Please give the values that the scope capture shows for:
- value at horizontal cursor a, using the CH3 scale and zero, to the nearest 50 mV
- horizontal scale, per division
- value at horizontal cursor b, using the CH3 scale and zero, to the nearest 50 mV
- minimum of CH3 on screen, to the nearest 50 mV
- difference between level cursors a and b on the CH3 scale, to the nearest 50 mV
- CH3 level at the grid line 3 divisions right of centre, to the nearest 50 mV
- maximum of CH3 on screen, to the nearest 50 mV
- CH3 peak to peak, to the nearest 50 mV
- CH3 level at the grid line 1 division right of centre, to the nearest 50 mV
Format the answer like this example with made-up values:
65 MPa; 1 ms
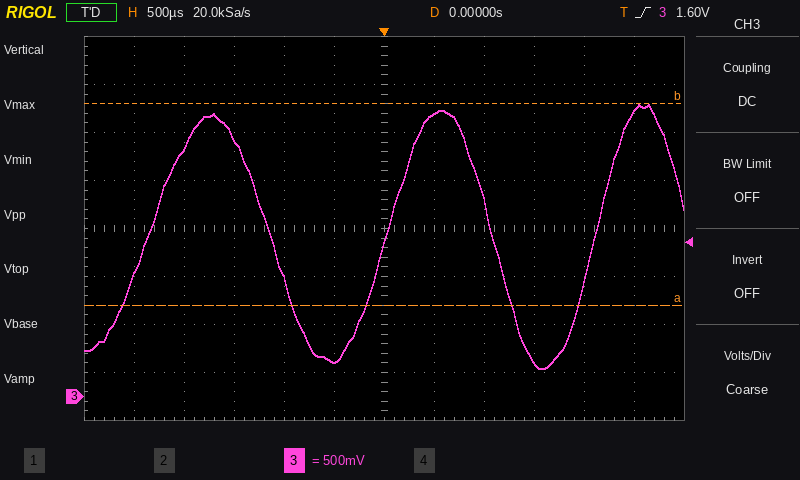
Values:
950 mV; 500 µs; 3.05 V; 300 mV; 2.10 V; 350 mV; 3.05 V; 2.75 V; 2.95 V
